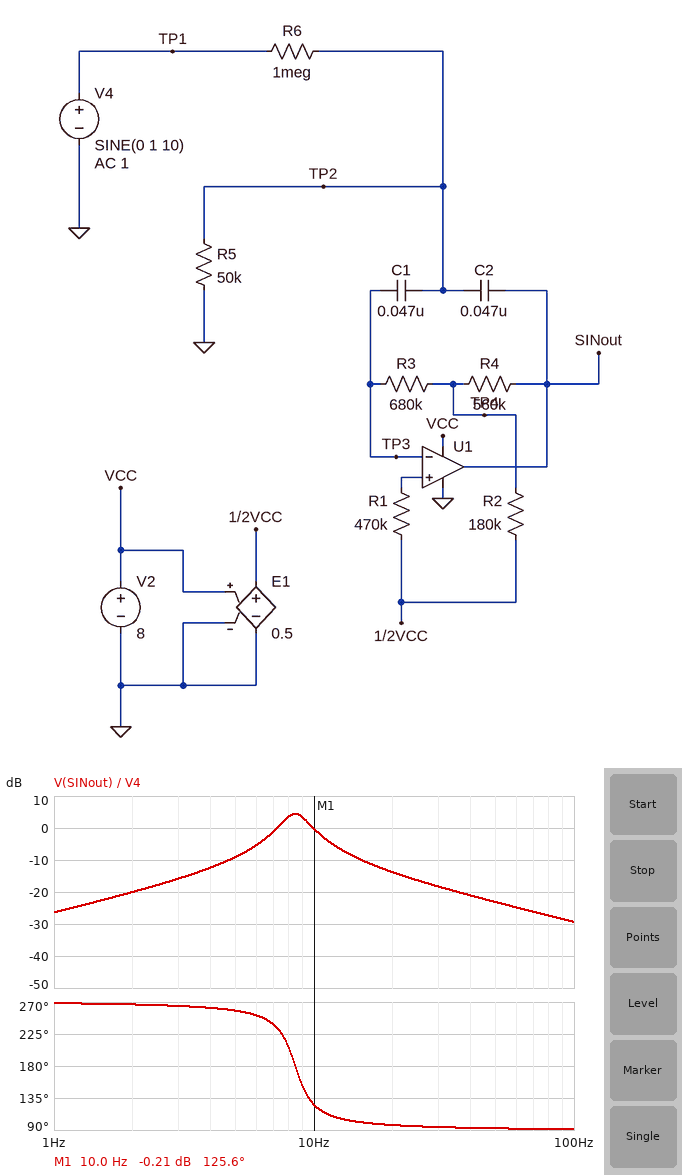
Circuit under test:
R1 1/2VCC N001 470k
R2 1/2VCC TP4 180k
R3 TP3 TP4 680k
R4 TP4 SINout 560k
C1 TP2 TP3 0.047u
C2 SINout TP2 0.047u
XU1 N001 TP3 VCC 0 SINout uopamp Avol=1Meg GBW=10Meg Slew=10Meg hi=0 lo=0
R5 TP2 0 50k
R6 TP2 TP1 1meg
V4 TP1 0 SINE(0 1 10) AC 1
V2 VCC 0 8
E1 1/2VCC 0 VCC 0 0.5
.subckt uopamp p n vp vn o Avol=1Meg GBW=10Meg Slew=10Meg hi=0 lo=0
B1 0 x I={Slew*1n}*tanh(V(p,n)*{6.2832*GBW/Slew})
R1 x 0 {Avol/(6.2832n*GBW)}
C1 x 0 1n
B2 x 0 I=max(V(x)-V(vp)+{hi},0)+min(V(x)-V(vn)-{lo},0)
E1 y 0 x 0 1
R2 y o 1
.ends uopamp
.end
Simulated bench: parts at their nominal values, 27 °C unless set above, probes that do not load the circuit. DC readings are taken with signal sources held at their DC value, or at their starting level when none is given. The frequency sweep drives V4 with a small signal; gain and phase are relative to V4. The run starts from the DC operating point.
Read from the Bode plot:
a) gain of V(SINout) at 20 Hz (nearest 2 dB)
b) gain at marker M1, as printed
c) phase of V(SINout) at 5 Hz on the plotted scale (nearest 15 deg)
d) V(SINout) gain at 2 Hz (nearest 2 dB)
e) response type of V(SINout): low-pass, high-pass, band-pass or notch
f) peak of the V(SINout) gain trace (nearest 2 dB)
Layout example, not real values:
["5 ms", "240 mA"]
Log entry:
["-14 dB", "-0.21 dB", "255 deg", "-20 dB", "band-pass", "4 dB"]
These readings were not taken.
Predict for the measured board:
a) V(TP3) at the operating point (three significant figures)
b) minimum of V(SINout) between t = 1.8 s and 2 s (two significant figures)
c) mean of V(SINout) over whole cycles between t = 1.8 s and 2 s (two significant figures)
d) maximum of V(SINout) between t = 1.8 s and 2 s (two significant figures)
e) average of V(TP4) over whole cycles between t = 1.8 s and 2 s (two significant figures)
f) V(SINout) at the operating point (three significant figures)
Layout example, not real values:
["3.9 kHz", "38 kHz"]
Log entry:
["4.00 V", "3.0 V", "4.0 V", "5.0 V", "4.0 V", "4.00 V"]
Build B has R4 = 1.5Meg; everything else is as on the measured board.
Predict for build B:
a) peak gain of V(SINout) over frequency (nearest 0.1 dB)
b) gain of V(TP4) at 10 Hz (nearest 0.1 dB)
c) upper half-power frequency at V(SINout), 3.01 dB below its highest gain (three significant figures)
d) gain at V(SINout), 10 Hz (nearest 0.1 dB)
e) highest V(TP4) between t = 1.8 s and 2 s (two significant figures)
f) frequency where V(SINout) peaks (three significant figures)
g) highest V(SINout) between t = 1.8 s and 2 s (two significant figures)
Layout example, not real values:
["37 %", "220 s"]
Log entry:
["11.9 dB", "-27.5 dB", "5.99 Hz", "-6.3 dB", "4.0 V", "5.54 Hz", "4.5 V"]
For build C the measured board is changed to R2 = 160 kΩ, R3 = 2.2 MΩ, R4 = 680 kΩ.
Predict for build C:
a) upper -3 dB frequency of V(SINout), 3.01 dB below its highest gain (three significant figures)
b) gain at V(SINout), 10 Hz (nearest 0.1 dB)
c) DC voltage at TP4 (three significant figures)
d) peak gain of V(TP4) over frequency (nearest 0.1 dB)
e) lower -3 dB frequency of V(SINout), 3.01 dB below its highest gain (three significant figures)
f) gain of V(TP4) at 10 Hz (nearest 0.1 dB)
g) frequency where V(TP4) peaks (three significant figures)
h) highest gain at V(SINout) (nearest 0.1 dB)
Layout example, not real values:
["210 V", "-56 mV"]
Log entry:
["4.72 Hz", "-7.5 dB", "4.00 V", "0.8 dB", "4.17 Hz", "-22.4 dB", "4.44 Hz", "15.7 dB"]
